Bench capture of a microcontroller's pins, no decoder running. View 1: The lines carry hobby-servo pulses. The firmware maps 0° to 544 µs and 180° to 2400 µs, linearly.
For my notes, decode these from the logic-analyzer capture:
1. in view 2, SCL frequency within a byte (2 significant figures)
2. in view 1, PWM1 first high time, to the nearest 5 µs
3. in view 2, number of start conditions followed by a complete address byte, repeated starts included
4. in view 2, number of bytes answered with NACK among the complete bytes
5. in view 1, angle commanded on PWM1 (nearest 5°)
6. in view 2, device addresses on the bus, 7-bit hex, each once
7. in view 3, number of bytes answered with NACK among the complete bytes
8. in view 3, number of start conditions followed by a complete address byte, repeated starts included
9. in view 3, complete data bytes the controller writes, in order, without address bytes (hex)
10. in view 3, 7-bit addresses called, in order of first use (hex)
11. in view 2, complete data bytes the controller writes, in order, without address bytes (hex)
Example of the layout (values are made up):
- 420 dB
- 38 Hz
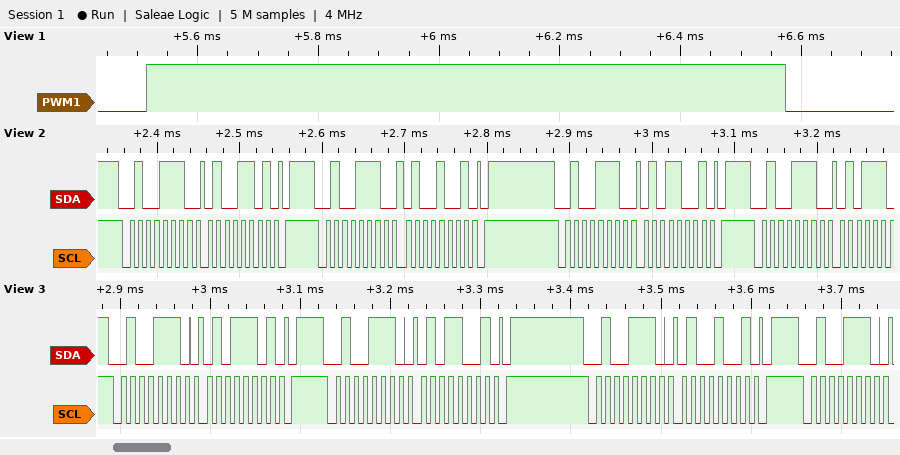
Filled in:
- 100 kHz
- 1060 µs
- 4
- 0
- 50°
- 0x27
- 0
- 4
- 5D 59 49
- 0x27
- 4D 49 59
